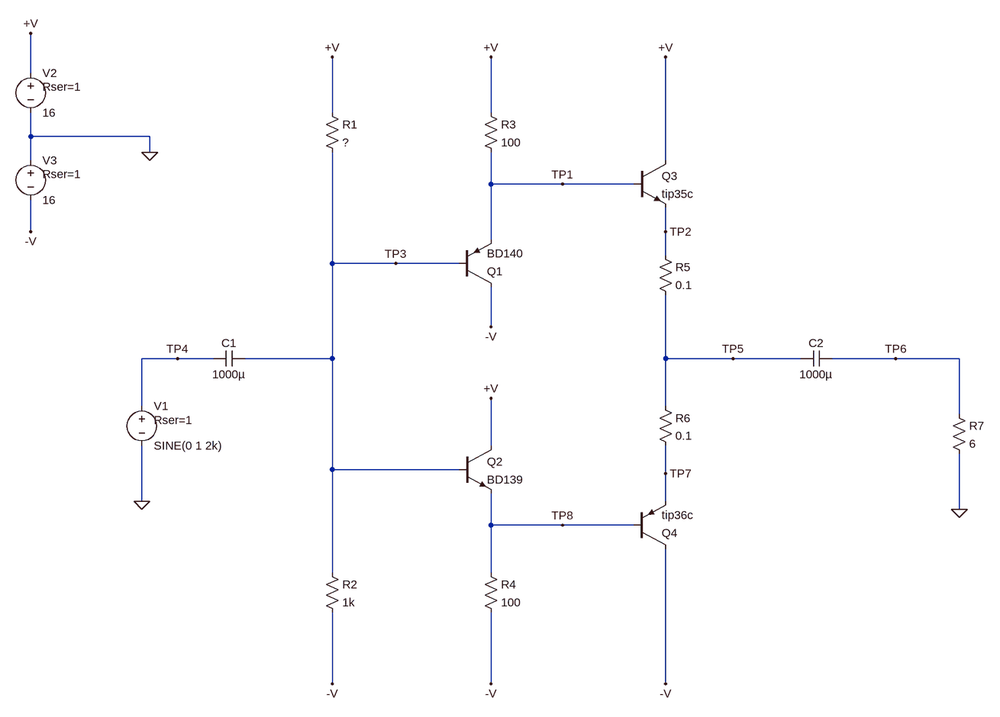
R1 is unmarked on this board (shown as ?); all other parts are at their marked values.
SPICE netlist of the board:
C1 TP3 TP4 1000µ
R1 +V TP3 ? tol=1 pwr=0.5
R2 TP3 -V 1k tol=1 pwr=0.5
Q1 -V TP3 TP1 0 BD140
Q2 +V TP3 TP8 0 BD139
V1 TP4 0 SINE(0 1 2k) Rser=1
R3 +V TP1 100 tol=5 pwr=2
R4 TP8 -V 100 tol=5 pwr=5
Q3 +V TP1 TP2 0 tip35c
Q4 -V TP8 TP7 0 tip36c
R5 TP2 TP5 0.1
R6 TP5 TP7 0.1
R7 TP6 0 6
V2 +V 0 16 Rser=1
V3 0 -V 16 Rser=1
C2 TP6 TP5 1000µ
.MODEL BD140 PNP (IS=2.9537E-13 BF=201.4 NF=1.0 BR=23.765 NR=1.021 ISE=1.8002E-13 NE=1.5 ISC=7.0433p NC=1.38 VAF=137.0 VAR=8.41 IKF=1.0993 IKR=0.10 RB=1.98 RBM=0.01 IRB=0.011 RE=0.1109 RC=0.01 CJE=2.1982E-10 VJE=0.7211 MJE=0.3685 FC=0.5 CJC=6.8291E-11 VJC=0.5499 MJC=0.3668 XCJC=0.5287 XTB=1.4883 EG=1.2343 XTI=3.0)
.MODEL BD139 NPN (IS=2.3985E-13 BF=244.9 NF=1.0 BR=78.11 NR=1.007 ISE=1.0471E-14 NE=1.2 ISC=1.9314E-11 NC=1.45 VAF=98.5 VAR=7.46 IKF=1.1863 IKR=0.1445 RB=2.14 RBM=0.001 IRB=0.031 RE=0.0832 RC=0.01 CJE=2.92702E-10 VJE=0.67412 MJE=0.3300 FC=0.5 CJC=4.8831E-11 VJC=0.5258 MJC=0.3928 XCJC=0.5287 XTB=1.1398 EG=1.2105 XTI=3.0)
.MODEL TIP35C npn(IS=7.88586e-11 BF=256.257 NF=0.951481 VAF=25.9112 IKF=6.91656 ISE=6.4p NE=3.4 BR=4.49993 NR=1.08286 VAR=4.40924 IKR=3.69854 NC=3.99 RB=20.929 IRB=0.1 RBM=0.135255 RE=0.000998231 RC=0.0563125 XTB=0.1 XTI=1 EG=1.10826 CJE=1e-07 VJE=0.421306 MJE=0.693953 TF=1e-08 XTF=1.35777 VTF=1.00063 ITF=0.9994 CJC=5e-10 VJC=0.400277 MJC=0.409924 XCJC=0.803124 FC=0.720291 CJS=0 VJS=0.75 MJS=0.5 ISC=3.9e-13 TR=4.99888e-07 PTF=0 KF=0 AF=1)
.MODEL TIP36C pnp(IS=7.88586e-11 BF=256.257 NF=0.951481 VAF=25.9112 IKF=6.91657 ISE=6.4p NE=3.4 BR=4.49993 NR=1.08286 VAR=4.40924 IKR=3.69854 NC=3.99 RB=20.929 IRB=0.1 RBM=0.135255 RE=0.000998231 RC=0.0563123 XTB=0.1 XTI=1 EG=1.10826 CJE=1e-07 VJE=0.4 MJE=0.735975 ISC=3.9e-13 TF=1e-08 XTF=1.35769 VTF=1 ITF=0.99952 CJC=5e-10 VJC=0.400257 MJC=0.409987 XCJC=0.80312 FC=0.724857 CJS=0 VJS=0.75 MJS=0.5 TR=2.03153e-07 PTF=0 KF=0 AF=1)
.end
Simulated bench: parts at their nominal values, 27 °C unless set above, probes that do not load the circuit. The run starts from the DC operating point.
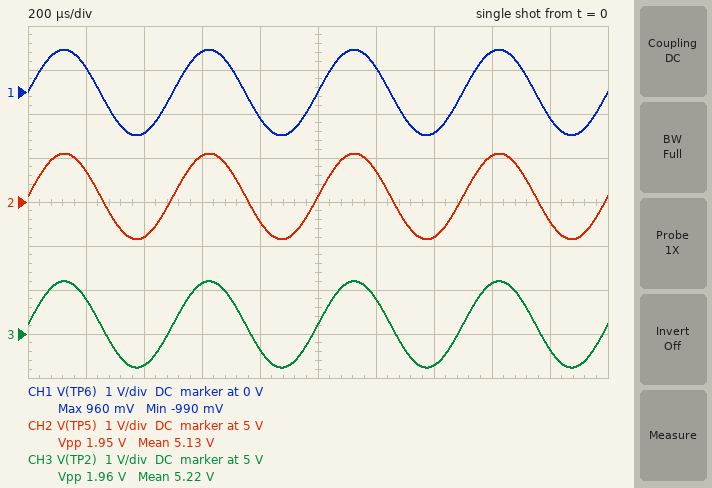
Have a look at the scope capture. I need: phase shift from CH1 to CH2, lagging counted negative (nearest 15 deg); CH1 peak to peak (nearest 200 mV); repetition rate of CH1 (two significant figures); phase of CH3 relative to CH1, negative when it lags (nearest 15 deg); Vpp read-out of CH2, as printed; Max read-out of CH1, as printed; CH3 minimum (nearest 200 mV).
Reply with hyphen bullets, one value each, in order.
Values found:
- 0 deg
- 2.0 V
- 2.0 kHz
- 0 deg
- 1.95 V
- 960 mV
- 4.2 V
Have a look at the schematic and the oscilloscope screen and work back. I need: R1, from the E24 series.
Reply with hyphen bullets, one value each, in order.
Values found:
- 470 Ω
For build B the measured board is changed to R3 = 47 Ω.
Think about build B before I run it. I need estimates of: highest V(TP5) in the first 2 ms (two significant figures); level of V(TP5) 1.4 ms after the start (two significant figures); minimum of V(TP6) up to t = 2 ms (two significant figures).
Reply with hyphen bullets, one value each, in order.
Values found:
- 6.2 V
- 4.3 V
- -990 mV
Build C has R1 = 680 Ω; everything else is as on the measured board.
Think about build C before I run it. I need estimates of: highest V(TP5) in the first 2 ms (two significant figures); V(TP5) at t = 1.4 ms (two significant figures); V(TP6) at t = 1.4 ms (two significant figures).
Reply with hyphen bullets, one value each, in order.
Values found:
- 3.7 V
- 1.8 V
- -930 mV
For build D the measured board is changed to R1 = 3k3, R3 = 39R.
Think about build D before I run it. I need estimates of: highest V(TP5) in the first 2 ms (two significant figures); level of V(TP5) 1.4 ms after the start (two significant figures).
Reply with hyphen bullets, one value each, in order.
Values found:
- -4.2 V
- -6.1 V
